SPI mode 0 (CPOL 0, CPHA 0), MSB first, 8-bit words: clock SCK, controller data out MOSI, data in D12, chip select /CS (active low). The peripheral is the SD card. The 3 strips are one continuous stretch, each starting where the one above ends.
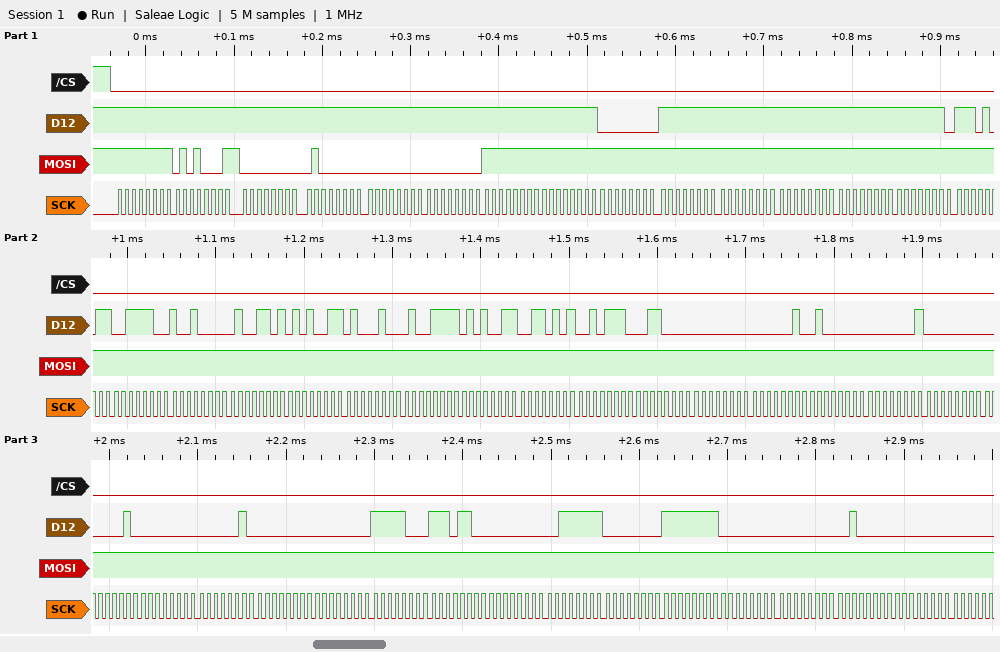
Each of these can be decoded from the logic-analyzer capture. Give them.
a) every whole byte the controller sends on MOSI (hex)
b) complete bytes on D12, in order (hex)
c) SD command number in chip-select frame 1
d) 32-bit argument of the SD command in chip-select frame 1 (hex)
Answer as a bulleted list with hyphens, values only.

- FF 51 00 40 00 00 FF FF FF FF FF FF FF FF FF FF FF FF FF FF FF FF FF FF FF FF FF FF FF FF FF FF FF FF FF FF FF FF FF FF FF FF FF FF FF
- FF FF FF FF FF FF FF FF 00 FF FF FF FF FE EB 3C 90 4D 53 44 4F 53 35 2E 30 00 02 40 01 00 02 00 02 00 00 F8 EC 00 3F 00 FF 00 00 20 00
- CMD17
- 0x00400000
